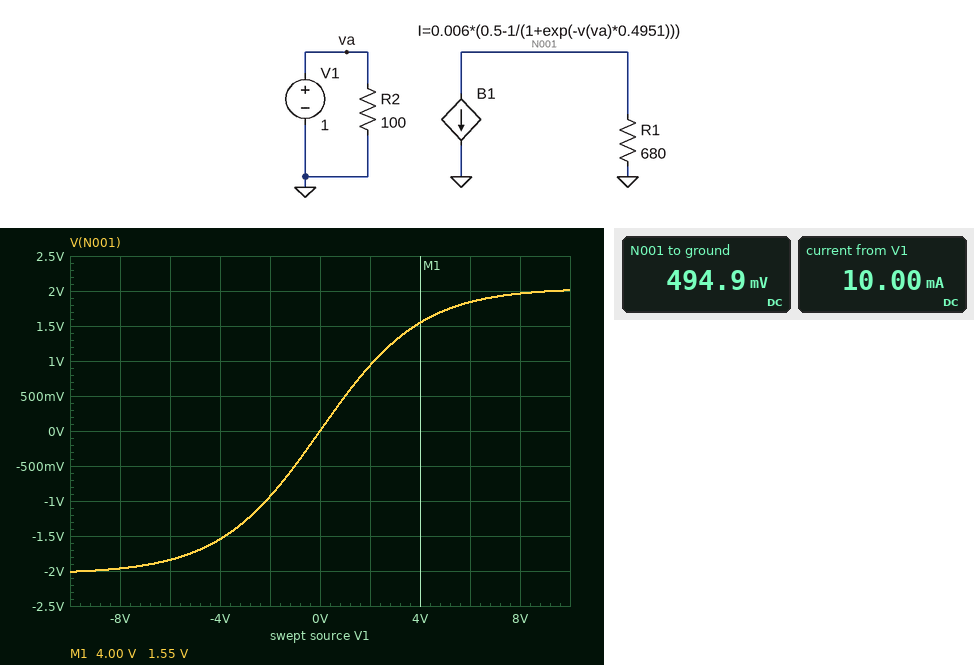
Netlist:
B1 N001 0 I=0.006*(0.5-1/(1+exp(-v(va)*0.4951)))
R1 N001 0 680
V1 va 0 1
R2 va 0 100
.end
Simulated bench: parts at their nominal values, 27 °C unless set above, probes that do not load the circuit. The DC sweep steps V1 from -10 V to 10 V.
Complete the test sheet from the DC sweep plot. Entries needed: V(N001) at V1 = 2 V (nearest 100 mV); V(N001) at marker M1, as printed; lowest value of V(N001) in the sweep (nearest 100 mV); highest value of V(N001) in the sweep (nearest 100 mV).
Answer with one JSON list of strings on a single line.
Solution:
["900 mV", "1.55 V", "-2.0 V", "2.0 V"]
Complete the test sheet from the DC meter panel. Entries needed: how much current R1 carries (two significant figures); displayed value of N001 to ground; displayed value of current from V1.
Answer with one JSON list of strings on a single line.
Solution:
["730 µA", "494.9 mV", "10.00 mA"]
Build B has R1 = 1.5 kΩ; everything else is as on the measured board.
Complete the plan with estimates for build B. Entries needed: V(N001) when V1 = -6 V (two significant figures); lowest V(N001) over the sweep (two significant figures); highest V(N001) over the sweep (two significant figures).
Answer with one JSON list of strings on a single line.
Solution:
["-4.1 V", "-4.4 V", "4.4 V"]
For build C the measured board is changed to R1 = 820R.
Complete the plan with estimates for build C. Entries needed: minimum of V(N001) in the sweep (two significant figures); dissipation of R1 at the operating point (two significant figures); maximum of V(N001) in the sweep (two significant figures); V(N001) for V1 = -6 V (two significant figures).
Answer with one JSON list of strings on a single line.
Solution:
["-2.4 V", "430 µW", "2.4 V", "-2.2 V"]
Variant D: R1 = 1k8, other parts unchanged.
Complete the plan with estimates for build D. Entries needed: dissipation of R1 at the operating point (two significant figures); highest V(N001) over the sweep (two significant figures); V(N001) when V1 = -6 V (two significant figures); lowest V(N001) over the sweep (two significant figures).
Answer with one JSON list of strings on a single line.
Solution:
["950 µW", "5.3 V", "-4.9 V", "-5.3 V"]
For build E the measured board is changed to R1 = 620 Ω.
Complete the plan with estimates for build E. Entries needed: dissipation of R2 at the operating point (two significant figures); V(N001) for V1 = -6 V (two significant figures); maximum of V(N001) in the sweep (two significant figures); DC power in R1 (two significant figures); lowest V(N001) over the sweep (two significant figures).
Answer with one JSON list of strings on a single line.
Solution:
["10 mW", "-1.7 V", "1.8 V", "330 µW", "-1.8 V"]
